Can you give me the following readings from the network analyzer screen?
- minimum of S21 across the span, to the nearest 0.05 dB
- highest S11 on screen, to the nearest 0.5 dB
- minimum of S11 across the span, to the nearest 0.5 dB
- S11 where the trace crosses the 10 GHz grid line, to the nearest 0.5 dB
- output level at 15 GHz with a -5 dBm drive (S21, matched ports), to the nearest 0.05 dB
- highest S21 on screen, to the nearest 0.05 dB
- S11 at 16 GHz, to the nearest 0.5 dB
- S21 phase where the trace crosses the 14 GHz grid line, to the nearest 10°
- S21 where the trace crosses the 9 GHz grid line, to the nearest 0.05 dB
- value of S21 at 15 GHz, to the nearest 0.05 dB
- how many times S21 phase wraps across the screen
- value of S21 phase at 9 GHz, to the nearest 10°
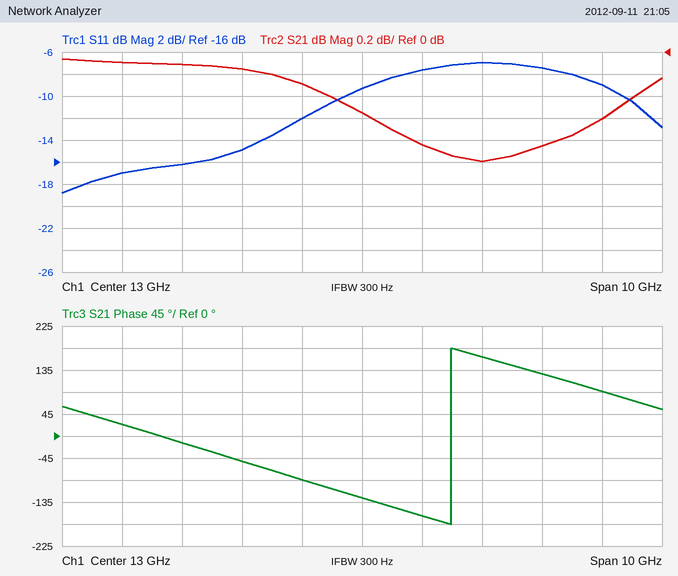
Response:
-1.00 dB
-7.0 dB
-19.0 dB
-16.0 dB
-6.00 dBm
-0.05 dB
-7.5 dB
-160°
-0.10 dB
-1.00 dB
1
20°
